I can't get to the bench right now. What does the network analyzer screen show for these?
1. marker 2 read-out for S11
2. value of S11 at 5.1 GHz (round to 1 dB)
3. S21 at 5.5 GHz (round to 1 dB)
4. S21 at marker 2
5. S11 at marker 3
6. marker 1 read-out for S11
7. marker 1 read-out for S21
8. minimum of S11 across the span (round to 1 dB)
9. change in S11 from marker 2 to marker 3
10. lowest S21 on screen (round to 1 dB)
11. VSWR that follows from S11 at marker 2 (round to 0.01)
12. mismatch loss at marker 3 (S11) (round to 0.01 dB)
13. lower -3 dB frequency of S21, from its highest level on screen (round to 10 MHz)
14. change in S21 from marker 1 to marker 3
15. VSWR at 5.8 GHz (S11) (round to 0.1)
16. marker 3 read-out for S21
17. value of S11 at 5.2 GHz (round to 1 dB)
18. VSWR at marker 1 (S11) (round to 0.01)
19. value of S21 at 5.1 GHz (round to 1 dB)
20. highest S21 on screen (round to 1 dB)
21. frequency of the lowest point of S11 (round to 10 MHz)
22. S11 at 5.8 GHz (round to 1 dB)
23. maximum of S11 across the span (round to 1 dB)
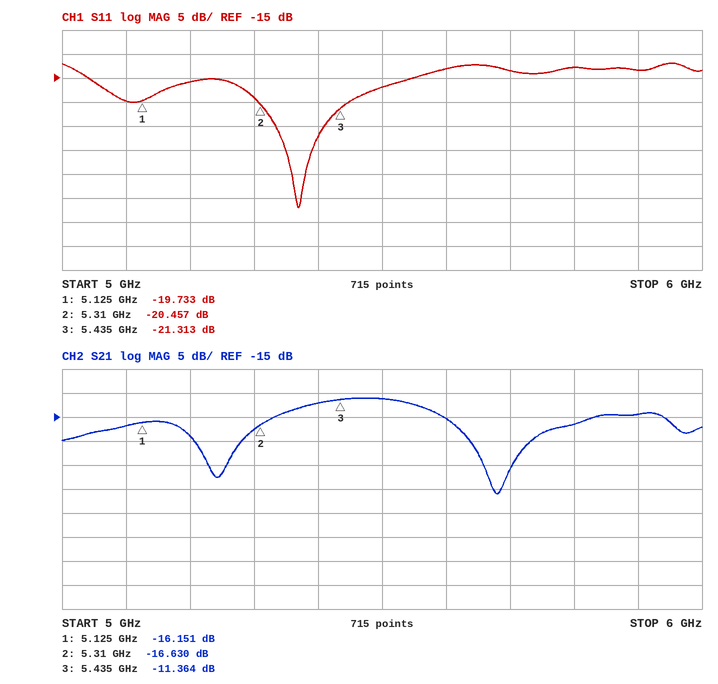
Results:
-20.457 dB
-20 dB
-11 dB
-16.630 dB
-21.313 dB
-19.733 dB
-16.151 dB
-42 dB
-0.856 dB
-31 dB
1.21
0.03 dB
5.35 GHz
4.787 dB
1.6
-11.364 dB
-16 dB
1.23
-17 dB
-11 dB
5.37 GHz
-13 dB
-12 dB
